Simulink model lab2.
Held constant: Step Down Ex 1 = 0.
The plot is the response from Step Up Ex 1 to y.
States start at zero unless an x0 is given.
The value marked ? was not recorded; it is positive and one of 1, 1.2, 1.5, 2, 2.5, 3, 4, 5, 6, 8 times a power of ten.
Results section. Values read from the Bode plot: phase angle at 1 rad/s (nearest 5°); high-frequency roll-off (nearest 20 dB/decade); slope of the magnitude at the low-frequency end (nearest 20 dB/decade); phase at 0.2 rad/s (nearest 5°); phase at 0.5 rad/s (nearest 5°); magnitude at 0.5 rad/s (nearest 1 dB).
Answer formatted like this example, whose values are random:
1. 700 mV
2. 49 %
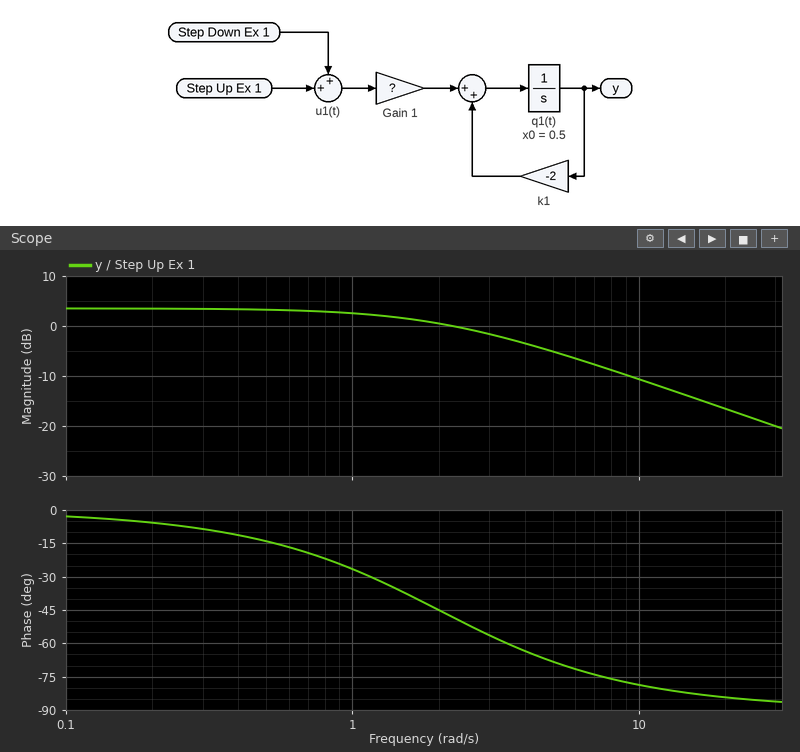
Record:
1. -25°
2. -20 dB/decade
3. 0 dB/decade
4. -5°
5. -15°
6. 3 dB
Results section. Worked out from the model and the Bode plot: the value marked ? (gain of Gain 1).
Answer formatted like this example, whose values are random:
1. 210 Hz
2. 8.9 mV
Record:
1. 3
